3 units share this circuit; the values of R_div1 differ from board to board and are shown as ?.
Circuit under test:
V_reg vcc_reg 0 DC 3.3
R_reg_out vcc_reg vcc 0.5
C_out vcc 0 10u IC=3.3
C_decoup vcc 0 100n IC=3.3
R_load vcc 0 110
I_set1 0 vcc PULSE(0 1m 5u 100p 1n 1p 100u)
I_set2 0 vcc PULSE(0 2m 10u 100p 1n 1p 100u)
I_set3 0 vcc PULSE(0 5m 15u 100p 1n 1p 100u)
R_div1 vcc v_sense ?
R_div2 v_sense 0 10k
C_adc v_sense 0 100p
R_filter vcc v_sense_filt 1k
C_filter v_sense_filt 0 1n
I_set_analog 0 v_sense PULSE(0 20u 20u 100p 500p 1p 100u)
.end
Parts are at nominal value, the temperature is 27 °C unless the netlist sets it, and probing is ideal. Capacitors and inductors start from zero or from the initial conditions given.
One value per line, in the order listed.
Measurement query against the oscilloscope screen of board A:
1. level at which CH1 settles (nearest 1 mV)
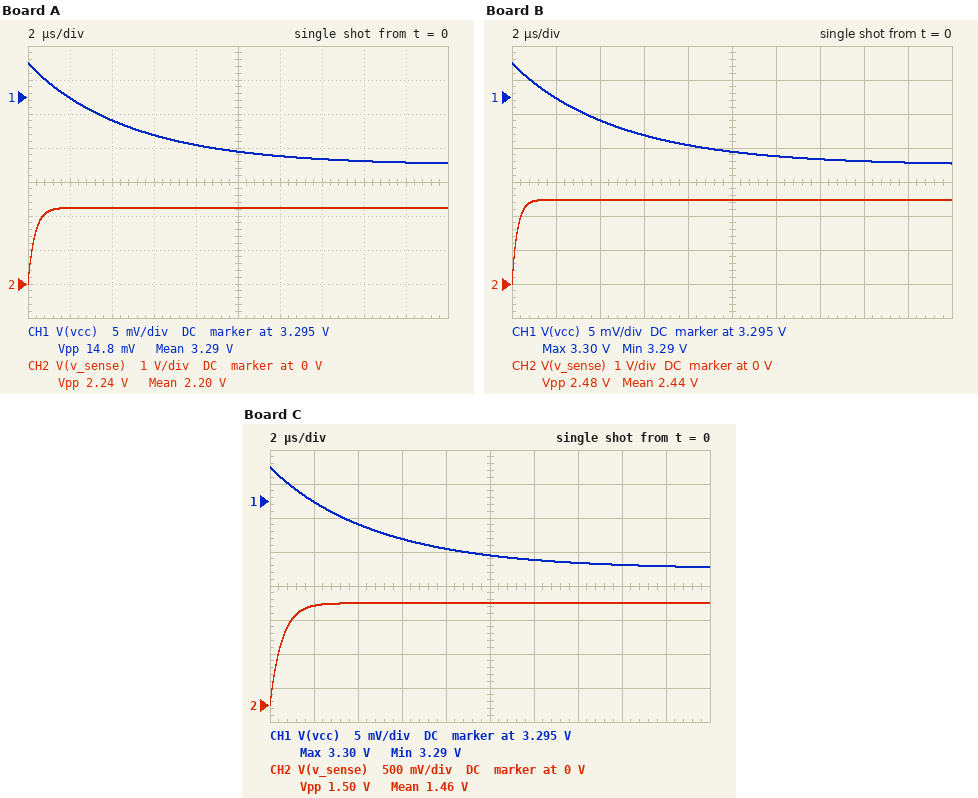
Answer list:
3.285 V
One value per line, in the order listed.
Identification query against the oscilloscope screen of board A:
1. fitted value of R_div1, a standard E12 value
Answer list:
4.7 kΩ
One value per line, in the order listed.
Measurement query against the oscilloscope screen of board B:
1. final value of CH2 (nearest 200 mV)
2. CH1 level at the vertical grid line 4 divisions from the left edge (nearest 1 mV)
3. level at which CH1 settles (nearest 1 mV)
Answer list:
2.4 V
3.288 V
3.285 V
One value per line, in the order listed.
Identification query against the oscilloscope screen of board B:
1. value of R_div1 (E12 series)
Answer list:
3.3 kΩ
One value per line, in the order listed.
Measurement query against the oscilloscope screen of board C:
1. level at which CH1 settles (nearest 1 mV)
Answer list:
3.285 V
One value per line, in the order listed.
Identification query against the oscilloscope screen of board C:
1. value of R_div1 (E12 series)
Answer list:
12 kΩ
